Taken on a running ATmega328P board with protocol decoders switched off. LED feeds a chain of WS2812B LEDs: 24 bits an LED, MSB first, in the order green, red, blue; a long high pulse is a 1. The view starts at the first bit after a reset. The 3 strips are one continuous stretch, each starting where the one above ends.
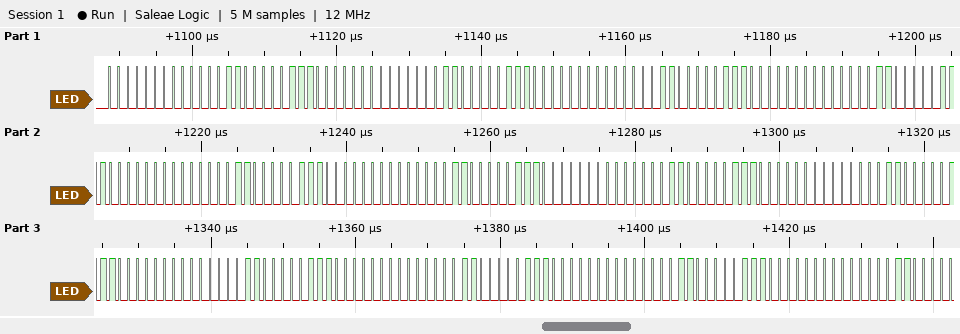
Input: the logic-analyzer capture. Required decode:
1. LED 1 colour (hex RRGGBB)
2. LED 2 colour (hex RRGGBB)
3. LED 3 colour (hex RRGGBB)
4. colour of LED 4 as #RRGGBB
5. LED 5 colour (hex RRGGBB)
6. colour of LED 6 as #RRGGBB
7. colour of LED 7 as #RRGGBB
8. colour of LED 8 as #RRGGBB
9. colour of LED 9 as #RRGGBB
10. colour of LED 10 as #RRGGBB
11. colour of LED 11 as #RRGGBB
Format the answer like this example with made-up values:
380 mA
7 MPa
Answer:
#06000E
#06000E
#06000E
#06000E
#06000E
#06000E
#06000E
#06000E
#06000E
#06000E
#06000E
